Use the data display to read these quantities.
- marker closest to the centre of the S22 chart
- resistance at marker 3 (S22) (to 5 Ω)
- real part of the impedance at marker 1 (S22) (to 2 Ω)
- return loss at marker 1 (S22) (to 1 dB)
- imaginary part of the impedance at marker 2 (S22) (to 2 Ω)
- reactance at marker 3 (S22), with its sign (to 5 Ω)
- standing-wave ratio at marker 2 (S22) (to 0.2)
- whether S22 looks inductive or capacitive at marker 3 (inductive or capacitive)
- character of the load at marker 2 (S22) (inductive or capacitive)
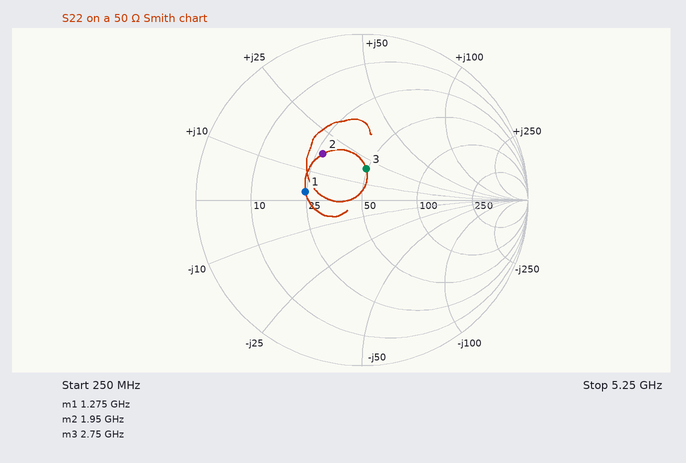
marker 3
50 Ω
24 Ω
9 dB
+18 Ω
+20 Ω
2.2
inductive
inductive
